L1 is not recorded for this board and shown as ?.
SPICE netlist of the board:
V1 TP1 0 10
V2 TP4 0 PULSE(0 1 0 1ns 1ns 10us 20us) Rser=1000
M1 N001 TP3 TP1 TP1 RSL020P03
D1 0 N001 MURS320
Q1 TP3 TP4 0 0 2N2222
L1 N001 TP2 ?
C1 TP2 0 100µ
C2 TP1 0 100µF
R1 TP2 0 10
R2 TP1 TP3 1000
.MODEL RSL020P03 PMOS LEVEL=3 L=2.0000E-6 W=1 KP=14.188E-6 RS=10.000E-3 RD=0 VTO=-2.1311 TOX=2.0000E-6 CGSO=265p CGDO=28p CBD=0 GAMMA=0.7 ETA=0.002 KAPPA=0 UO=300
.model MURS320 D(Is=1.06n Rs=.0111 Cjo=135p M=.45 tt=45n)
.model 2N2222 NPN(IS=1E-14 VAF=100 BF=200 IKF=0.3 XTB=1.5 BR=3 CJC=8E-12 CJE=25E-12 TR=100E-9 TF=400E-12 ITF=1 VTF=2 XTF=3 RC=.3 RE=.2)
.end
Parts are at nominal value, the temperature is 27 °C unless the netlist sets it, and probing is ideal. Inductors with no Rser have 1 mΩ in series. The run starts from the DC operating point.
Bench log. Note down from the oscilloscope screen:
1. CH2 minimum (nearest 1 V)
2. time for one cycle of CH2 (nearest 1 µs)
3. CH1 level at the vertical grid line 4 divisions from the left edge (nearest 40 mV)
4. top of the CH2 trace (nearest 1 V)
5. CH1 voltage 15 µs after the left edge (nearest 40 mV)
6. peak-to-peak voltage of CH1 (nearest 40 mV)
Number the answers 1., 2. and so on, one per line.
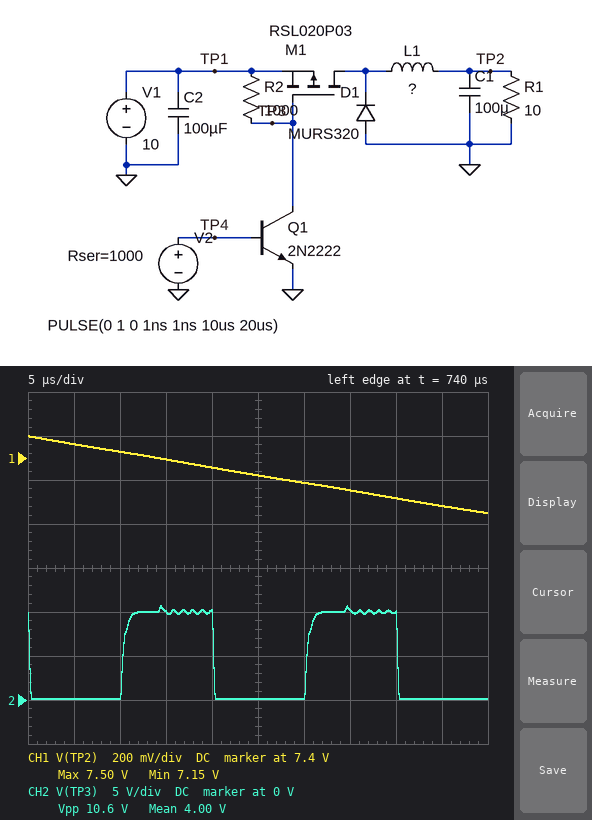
1. 0 V
2. 20 µs
3. 7.36 V
4. 11 V
5. 7.40 V
6. 360 mV
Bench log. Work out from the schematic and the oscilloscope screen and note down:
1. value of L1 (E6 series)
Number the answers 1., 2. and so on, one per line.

1. 330 µH
